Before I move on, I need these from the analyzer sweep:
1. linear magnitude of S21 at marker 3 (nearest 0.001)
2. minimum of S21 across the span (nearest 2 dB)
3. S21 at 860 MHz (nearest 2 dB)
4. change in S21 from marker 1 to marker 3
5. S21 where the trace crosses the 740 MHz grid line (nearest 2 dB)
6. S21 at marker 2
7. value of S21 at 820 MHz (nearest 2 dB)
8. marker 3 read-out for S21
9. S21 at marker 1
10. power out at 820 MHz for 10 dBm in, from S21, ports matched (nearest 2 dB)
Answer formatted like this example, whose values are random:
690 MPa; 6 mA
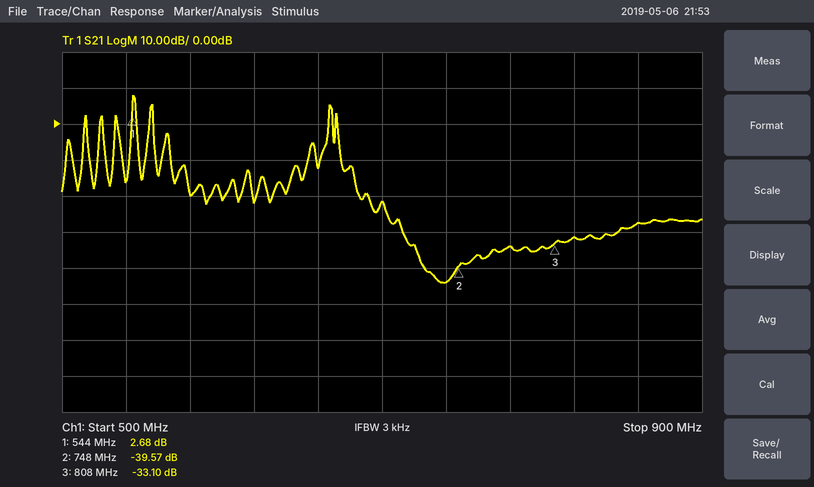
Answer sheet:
0.022; -44 dB; -28 dB; -35.78 dB; -44 dB; -39.57 dB; -32 dB; -33.10 dB; 2.68 dB; -22 dBm
